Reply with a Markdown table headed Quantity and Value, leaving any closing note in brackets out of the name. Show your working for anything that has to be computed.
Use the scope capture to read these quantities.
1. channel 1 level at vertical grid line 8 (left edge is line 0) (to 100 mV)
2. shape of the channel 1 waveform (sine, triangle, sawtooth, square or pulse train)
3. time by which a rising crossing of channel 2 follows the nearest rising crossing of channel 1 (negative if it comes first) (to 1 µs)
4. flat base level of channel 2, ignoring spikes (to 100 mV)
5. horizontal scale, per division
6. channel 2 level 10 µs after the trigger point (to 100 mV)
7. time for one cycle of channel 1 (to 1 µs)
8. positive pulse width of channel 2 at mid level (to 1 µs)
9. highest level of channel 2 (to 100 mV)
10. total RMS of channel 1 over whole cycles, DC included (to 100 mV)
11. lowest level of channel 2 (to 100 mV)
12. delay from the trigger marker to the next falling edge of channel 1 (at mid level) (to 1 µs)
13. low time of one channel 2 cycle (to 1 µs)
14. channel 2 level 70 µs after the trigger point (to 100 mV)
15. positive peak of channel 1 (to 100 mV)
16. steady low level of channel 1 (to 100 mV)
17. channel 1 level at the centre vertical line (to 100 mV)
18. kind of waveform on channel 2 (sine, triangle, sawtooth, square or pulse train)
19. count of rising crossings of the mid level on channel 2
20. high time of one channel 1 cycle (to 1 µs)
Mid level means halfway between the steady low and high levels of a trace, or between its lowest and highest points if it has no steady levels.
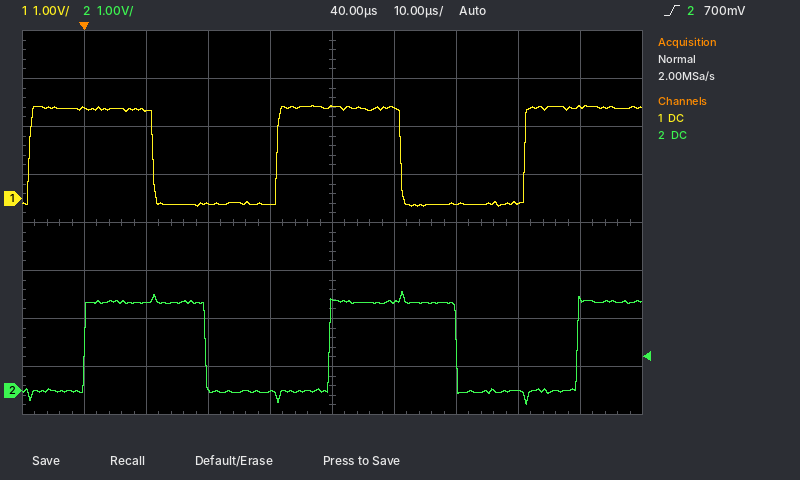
| Quantity | Value |
|---|---|
| channel 1 level at vertical grid line 8 (left edge is line 0) | -100 mV |
| shape of the channel 1 waveform | square |
| time by which a rising crossing of channel 2 follows the nearest rising crossing of channel 1 (negative if it comes first) | +9 µs |
| flat base level of channel 2, ignoring spikes | 0.0 V |
| horizontal scale, per division | 10 µs |
| channel 2 level 10 µs after the trigger point | 1.8 V |
| time for one cycle of channel 1 | 40 µs |
| positive pulse width of channel 2 at mid level | 20 µs |
| highest level of channel 2 | 2.1 V |
| total RMS of channel 1 over whole cycles, DC included | √(0.5 × (1.9 V)² + 0.5 × (-100 mV)²) ≈ 1.3 V |
| lowest level of channel 2 | -300 mV |
| delay from the trigger marker to the next falling edge of channel 1 (at mid level) | 11 µs |
| low time of one channel 2 cycle | 20 µs |
| channel 2 level 70 µs after the trigger point | 0.0 V |
| positive peak of channel 1 | 1.9 V |
| steady low level of channel 1 | -100 mV |
| channel 1 level at the centre vertical line | 1.9 V |
| kind of waveform on channel 2 | square |
| count of rising crossings of the mid level on channel 2 | 3 |
| high time of one channel 1 cycle | 20 µs |
